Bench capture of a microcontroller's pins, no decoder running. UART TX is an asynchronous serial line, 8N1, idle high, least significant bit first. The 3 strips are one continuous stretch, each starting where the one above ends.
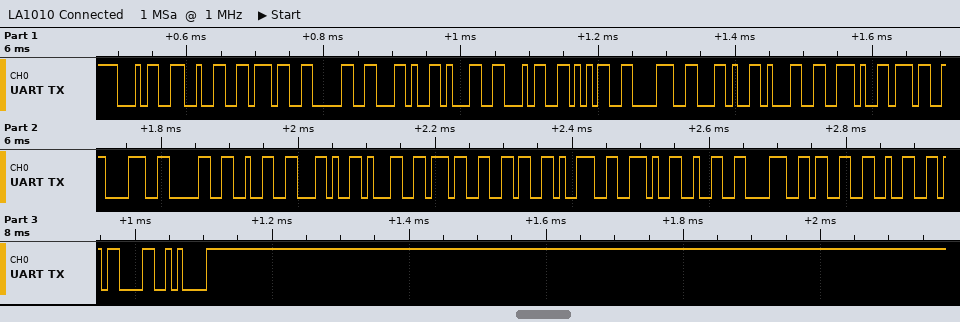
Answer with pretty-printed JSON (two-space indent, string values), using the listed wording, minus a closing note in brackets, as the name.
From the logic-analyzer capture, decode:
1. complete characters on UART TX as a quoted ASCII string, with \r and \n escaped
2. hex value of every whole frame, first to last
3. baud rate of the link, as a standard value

{
  "complete characters on UART TX as a quoted ASCII string, with \\r and \\n escaped": "\"4270,1458,1.7802,1769.2832\\r\\n\"",
  "hex value of every whole frame, first to last": "0x34 0x32 0x37 0x30 0x2C 0x31 0x34 0x35 0x38 0x2C 0x31 0x2E 0x37 0x38 0x30 0x32 0x2C 0x31 0x37 0x36 0x39 0x2E 0x32 0x38 0x33 0x32 0x0D 0x0A",
  "baud rate of the link, as a standard value": "115200 baud"
}
